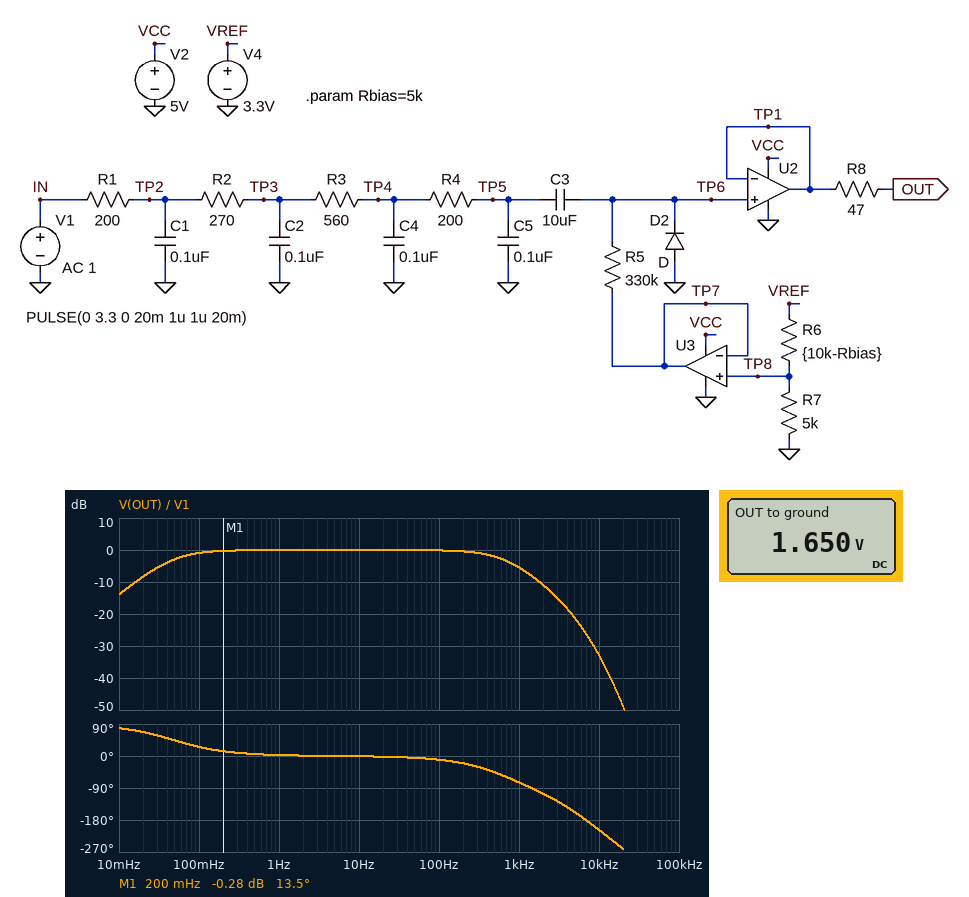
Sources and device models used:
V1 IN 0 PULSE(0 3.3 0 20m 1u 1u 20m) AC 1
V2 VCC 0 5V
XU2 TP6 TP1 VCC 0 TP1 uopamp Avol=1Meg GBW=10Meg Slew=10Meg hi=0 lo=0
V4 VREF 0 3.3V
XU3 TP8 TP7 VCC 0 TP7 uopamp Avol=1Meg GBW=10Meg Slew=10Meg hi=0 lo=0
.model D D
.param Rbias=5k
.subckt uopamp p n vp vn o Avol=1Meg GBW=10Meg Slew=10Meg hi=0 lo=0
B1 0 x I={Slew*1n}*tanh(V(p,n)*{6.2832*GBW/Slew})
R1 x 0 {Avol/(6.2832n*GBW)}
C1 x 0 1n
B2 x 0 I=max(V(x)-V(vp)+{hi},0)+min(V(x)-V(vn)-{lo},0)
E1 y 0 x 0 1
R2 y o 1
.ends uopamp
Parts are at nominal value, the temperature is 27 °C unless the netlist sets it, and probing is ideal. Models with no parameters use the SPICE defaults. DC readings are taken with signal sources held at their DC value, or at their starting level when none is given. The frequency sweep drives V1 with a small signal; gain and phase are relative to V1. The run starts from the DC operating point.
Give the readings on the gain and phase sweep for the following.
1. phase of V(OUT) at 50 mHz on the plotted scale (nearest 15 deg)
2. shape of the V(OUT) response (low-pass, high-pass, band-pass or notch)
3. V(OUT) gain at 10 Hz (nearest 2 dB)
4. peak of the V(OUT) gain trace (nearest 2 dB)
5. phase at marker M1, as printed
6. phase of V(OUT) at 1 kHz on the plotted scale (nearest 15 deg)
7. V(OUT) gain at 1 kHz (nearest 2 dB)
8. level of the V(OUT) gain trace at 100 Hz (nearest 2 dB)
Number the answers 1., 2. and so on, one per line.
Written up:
1. 45 deg
2. band-pass
3. 0 dB
4. 0 dB
5. 13.5 deg
6. -75 deg
7. -6 dB
8. 0 dB
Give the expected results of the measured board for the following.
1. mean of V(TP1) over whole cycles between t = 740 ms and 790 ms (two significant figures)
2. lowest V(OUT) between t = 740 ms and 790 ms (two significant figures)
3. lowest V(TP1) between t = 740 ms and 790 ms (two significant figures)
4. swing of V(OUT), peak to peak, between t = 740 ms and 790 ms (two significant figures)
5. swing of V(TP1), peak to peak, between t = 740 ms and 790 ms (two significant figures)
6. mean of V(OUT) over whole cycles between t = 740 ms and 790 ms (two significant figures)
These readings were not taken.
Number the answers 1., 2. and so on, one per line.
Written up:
1. 3.0 V
2. 1.5 V
3. 1.5 V
4. 3.1 V
5. 3.1 V
6. 3.0 V
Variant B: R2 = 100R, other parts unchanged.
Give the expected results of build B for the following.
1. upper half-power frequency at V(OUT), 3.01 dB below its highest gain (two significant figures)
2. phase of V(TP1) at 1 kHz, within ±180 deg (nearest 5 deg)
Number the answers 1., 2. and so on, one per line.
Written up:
1. 780 Hz
2. -65 deg
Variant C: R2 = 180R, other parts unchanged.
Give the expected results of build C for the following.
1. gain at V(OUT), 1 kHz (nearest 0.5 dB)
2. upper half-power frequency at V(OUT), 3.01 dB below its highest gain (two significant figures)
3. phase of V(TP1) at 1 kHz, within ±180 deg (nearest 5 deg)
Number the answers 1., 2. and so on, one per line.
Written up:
1. -5.0 dB
2. 710 Hz
3. -70 deg
